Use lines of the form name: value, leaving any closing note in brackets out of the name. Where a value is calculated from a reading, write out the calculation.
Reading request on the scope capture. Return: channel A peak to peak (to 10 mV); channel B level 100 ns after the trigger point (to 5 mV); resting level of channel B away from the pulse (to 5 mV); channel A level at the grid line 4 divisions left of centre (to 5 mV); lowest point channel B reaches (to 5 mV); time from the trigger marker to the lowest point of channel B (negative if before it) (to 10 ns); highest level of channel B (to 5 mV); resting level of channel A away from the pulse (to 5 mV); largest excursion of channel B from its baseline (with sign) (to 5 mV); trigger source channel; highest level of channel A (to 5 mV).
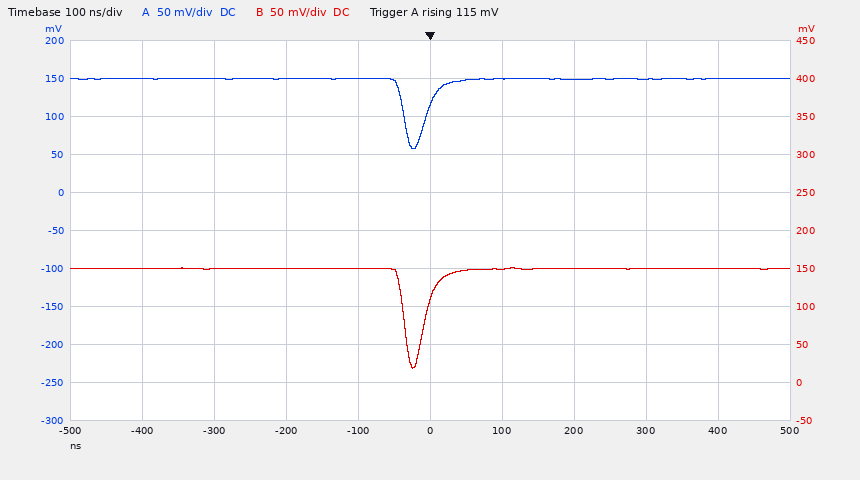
channel A peak to peak: 90 mV
channel B level 100 ns after the trigger point: 150 mV
resting level of channel B away from the pulse: 150 mV
channel A level at the grid line 4 divisions left of centre: 150 mV
lowest point channel B reaches: 20 mV
time from the trigger marker to the lowest point of channel B (negative if before it): -20 ns
highest level of channel B: 150 mV
resting level of channel A away from the pulse: 150 mV
largest excursion of channel B from its baseline (with sign): 20 mV − (150 mV) = -130 mV
trigger source channel: channel A
highest level of channel A: 150 mV
